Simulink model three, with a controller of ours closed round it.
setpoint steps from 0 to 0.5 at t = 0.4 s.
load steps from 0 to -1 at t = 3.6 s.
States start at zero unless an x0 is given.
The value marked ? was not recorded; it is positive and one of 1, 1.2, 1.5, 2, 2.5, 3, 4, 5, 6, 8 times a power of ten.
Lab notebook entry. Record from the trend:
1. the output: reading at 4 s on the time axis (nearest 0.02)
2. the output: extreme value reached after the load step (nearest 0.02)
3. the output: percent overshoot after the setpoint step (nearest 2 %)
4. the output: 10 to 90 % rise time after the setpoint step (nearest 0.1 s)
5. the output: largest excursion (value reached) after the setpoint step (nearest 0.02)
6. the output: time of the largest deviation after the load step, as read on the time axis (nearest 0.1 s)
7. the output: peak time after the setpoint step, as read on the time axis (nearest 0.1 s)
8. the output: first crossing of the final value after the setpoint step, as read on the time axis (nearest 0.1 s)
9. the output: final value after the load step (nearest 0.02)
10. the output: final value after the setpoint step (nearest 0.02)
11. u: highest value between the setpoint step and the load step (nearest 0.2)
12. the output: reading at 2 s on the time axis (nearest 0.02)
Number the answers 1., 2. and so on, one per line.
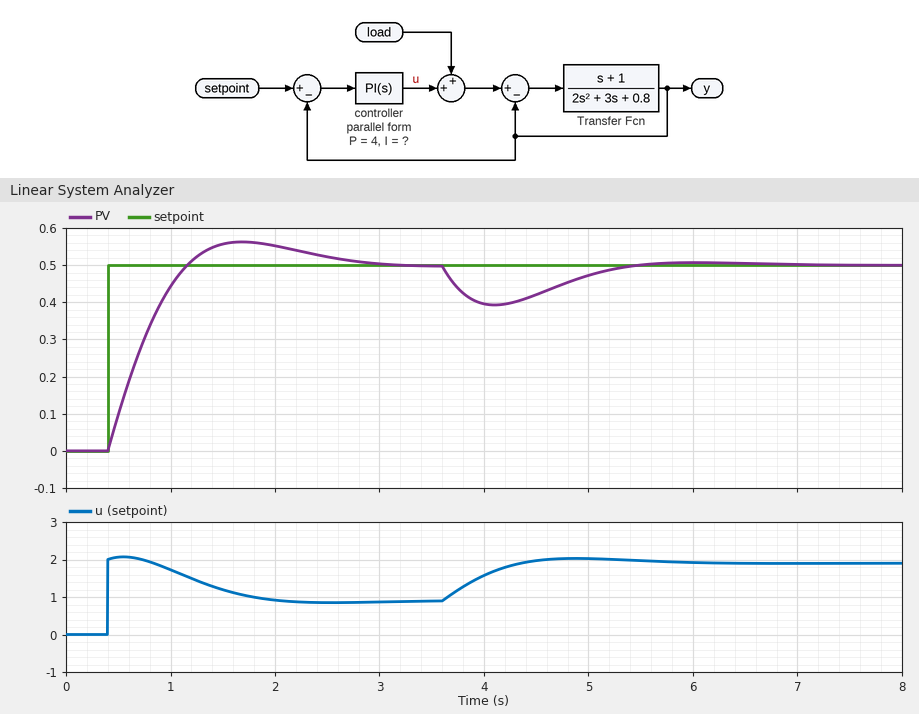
1. 0.40
2. 0.40
3. 12 %
4. 0.6 s
5. 0.56
6. 4.1 s
7. 1.7 s
8. 1.2 s
9. 0.50
10. 0.50
11. 2.0
12. 0.56
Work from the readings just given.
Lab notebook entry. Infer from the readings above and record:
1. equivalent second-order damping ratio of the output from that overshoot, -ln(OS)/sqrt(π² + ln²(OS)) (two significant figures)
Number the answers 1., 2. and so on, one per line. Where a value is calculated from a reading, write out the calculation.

1. ln(0.12) = -2.120; 2.120 / sqrt(9.870 + 4.496) = 0.56
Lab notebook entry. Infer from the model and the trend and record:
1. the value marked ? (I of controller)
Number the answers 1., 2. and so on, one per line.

1. 10
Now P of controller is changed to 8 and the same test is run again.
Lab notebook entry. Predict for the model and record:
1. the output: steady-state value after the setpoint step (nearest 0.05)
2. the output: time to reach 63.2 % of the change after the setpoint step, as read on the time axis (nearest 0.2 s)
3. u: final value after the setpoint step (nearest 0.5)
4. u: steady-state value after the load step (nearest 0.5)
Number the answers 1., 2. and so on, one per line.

1. 0.50
2. 0.6 s
3. 1.0
4. 2.0
